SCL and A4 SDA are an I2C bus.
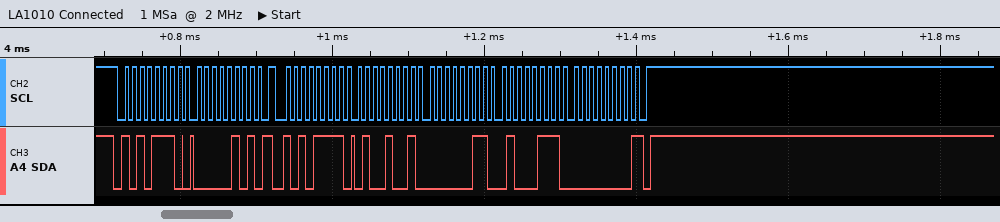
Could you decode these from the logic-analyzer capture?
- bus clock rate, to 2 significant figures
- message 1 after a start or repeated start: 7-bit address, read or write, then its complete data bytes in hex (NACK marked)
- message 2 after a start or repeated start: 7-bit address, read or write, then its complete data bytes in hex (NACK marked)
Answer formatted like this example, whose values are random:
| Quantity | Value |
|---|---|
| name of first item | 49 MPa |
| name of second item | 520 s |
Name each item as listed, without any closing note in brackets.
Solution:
| Quantity | Value |
|---|---|
| bus clock rate, to 2 significant figures | 100 kHz |
| message 1 after a start or repeated start: 7-bit address, read or write, then its complete data bytes in hex | 0x57 write: 05 |
| message 2 after a start or repeated start: 7-bit address, read or write, then its complete data bytes in hex | 0x57 read: 49 03 47 00 NACK |
